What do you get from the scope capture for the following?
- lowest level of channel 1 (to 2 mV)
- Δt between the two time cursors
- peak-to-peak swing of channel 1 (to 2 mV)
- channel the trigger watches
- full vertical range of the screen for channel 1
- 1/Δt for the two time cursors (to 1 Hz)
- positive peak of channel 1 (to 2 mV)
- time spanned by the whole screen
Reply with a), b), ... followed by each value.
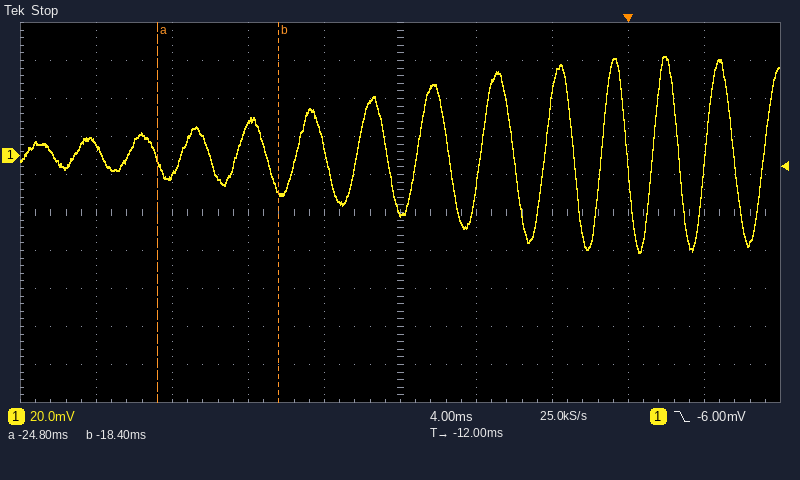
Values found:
a) -52 mV
b) 6.4 ms
c) 104 mV
d) channel 1
e) 200 mV
f) 156 Hz
g) 52 mV
h) 40 ms
